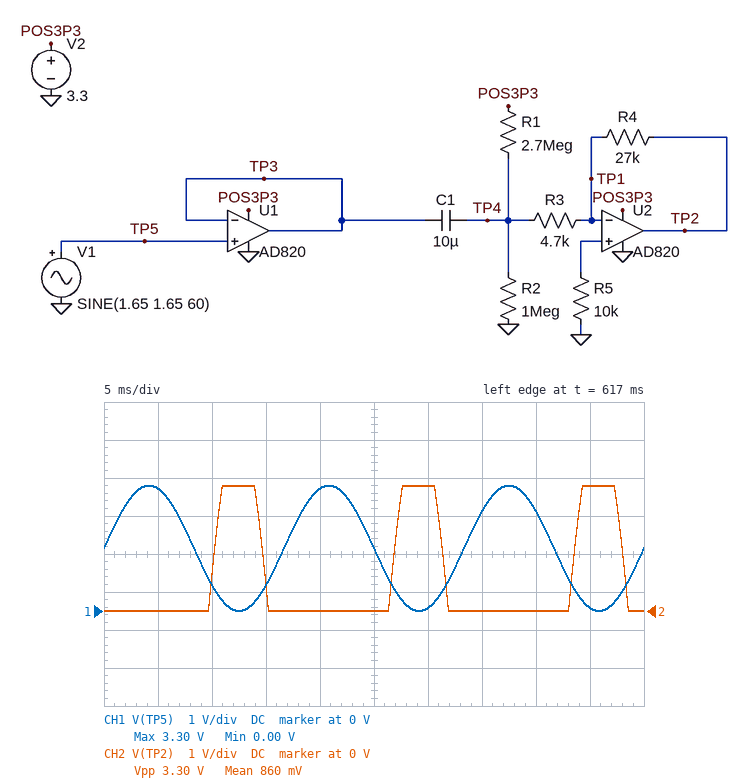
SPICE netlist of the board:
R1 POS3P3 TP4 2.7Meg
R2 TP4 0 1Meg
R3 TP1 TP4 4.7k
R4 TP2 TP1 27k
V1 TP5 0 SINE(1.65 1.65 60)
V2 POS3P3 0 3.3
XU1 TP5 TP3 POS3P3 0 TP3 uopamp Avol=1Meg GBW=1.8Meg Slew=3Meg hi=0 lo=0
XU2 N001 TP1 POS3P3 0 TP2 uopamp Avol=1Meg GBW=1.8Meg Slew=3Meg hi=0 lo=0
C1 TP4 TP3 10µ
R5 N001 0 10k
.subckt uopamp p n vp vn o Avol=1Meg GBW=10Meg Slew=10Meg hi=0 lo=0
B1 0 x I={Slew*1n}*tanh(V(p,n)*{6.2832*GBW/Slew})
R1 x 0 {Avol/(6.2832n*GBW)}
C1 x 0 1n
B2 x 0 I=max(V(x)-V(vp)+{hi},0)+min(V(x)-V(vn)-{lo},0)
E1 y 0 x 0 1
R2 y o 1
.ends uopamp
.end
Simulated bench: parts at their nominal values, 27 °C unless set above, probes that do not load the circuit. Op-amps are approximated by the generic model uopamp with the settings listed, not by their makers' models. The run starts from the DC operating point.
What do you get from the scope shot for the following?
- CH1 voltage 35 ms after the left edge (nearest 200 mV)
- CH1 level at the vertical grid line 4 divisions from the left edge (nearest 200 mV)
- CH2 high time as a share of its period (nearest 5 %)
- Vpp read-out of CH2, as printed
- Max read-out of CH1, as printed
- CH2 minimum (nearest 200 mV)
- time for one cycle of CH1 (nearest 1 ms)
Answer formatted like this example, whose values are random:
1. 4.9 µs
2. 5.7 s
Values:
1. 2.6 V
2. 3.2 V
3. 25 %
4. 3.30 V
5. 3.30 V
6. 0 V
7. 17 ms
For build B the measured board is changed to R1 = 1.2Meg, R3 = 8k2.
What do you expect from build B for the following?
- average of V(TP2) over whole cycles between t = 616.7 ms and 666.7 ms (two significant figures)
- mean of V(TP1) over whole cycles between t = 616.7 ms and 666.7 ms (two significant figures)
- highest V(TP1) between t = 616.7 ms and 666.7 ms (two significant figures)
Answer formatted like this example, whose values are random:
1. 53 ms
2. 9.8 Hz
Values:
1. 700 mV
2. 720 mV
3. 1.8 V
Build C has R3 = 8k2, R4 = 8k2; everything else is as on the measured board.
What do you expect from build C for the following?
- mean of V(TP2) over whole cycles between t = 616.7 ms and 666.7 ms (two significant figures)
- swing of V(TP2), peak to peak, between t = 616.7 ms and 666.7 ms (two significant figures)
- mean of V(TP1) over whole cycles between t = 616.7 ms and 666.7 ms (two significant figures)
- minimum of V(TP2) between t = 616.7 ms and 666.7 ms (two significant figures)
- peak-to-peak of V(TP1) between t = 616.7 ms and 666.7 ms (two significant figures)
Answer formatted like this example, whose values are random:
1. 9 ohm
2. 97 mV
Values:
1. 350 mV
2. 1.3 V
3. 360 mV
4. -2.9 mV
5. 1.0 V
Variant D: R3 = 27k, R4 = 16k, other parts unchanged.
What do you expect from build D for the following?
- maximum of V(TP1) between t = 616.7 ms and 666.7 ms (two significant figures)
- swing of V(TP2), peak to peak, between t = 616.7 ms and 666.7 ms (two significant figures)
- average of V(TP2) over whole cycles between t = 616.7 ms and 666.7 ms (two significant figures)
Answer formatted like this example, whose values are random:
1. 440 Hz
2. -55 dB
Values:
1. 700 mV
2. 840 mV
3. 240 mV
